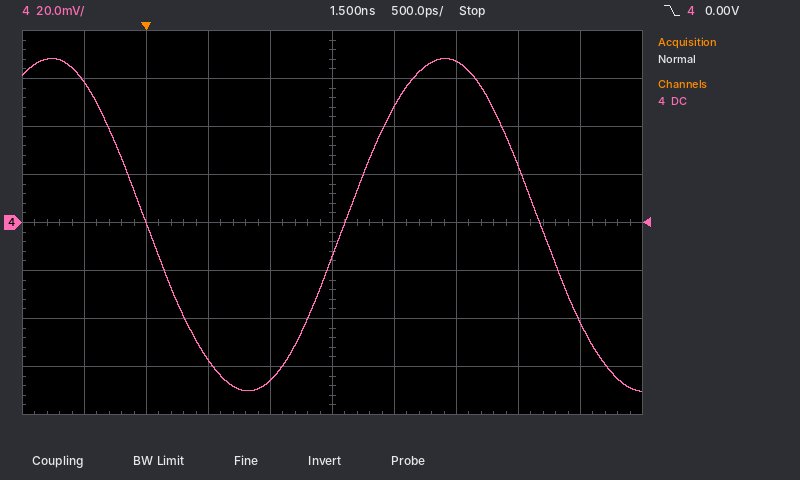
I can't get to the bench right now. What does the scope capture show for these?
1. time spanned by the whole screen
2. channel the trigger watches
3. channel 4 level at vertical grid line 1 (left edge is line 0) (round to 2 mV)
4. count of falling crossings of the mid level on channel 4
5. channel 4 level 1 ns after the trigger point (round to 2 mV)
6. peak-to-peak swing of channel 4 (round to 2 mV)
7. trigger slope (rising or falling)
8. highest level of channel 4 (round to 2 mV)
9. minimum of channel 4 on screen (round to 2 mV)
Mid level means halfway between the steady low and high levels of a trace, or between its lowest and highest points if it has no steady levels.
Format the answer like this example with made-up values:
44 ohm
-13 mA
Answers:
5 ns
channel 4
58 mV
2
-66 mV
138 mV
falling
68 mV
-70 mV
